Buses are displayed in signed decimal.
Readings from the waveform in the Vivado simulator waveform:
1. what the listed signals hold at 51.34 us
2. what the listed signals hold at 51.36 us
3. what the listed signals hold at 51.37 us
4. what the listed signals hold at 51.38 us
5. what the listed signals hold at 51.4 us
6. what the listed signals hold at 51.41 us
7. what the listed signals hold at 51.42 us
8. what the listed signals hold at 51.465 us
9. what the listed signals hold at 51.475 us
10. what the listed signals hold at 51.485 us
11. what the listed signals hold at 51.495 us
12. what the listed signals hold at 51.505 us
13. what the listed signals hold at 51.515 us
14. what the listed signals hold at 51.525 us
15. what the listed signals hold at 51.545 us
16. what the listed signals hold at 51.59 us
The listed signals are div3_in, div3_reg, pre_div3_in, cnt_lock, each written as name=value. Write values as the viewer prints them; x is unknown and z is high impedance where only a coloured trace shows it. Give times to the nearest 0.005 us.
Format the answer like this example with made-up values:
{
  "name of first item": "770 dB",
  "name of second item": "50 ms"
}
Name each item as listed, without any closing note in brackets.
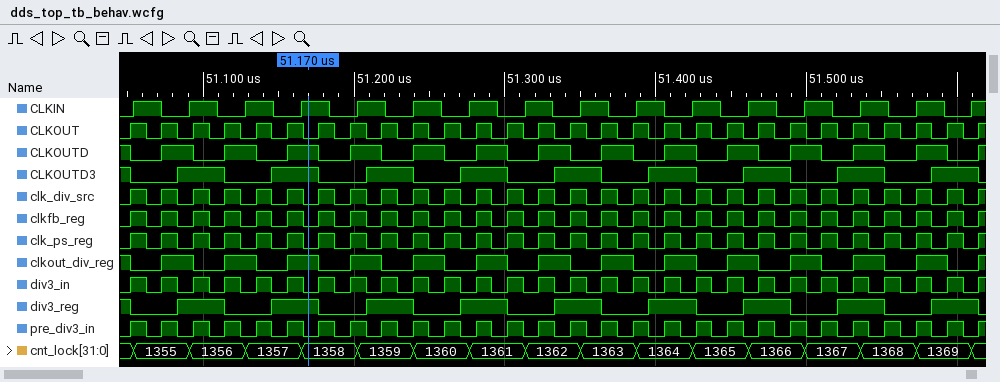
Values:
{
  "what the listed signals hold at 51.34 us": "div3_in=0, div3_reg=1, pre_div3_in=0, cnt_lock=1362",
  "what the listed signals hold at 51.36 us": "div3_in=0, div3_reg=1, pre_div3_in=0, cnt_lock=1363",
  "what the listed signals hold at 51.37 us": "div3_in=1, div3_reg=0, pre_div3_in=1, cnt_lock=1363",
  "what the listed signals hold at 51.38 us": "div3_in=0, div3_reg=0, pre_div3_in=0, cnt_lock=1363",
  "what the listed signals hold at 51.4 us": "div3_in=0, div3_reg=1, pre_div3_in=0, cnt_lock=1364",
  "what the listed signals hold at 51.41 us": "div3_in=1, div3_reg=1, pre_div3_in=1, cnt_lock=1364",
  "what the listed signals hold at 51.42 us": "div3_in=0, div3_reg=1, pre_div3_in=0, cnt_lock=1364",
  "what the listed signals hold at 51.465 us": "div3_in=0, div3_reg=1, pre_div3_in=0, cnt_lock=1366",
  "what the listed signals hold at 51.475 us": "div3_in=1, div3_reg=1, pre_div3_in=1, cnt_lock=1366",
  "what the listed signals hold at 51.485 us": "div3_in=0, div3_reg=1, pre_div3_in=0, cnt_lock=1366",
  "what the listed signals hold at 51.495 us": "div3_in=1, div3_reg=0, pre_div3_in=1, cnt_lock=1366",
  "what the listed signals hold at 51.505 us": "div3_in=0, div3_reg=0, pre_div3_in=0, cnt_lock=1367",
  "what the listed signals hold at 51.515 us": "div3_in=1, div3_reg=0, pre_div3_in=1, cnt_lock=1367",
  "what the listed signals hold at 51.525 us": "div3_in=0, div3_reg=1, pre_div3_in=0, cnt_lock=1367",
  "what the listed signals hold at 51.545 us": "div3_in=0, div3_reg=1, pre_div3_in=0, cnt_lock=1368",
  "what the listed signals hold at 51.59 us": "div3_in=0, div3_reg=1, pre_div3_in=0, cnt_lock=1369"
}
